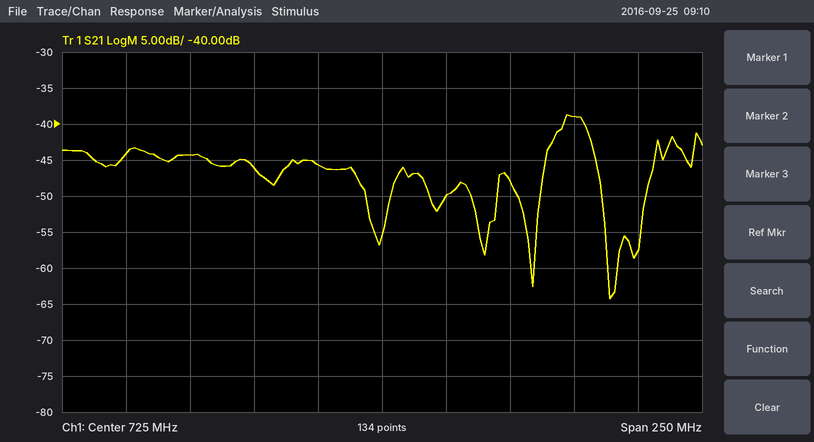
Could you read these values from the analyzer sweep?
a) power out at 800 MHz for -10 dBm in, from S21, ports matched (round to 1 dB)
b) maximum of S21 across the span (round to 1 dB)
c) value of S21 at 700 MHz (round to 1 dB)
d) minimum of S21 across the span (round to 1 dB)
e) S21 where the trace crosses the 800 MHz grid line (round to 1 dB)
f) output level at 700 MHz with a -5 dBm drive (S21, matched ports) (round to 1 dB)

-49 dBm
-39 dB
-46 dB
-64 dB
-39 dB
-51 dBm
